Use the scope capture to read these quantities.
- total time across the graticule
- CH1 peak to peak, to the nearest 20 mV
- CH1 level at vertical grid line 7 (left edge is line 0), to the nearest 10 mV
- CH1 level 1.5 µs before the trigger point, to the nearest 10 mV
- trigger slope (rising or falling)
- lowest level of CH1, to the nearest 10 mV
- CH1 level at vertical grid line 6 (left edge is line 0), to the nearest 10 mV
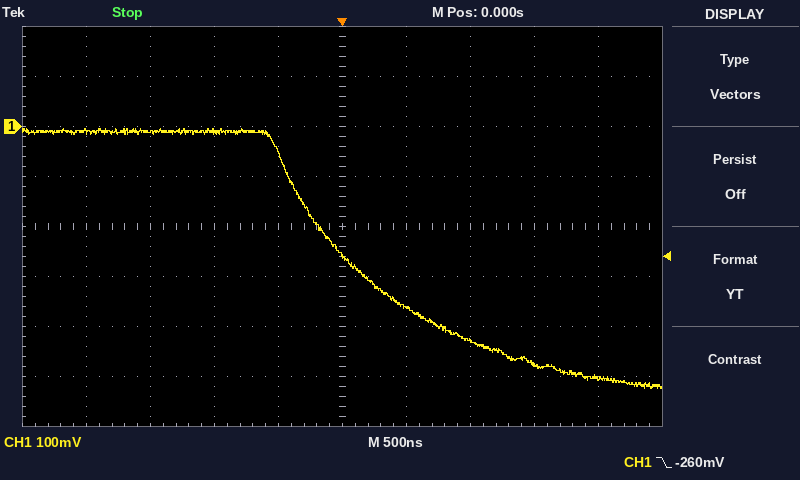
5 µs
520 mV
-430 mV
-10 mV
falling
-520 mV
-360 mV
